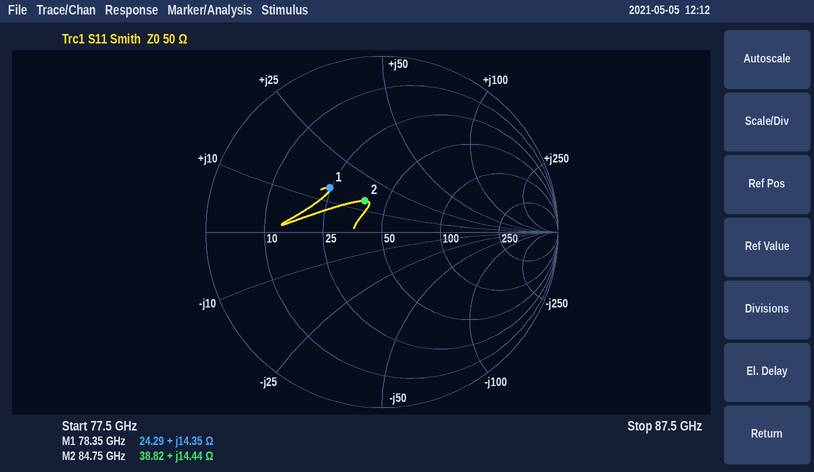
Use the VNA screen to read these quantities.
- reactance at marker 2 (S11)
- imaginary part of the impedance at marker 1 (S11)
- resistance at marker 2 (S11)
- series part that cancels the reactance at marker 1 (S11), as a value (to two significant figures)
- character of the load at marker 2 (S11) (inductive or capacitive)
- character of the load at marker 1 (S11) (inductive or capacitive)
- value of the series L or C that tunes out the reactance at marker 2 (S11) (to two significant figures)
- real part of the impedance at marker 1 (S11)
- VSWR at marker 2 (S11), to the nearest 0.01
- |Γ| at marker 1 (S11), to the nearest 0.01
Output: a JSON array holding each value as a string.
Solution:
["+14.44 Ω", "+14.35 Ω", "38.82 Ω", "140 fF", "inductive", "inductive", "130 fF", "24.29 Ω", "1.51", "0.39"]
